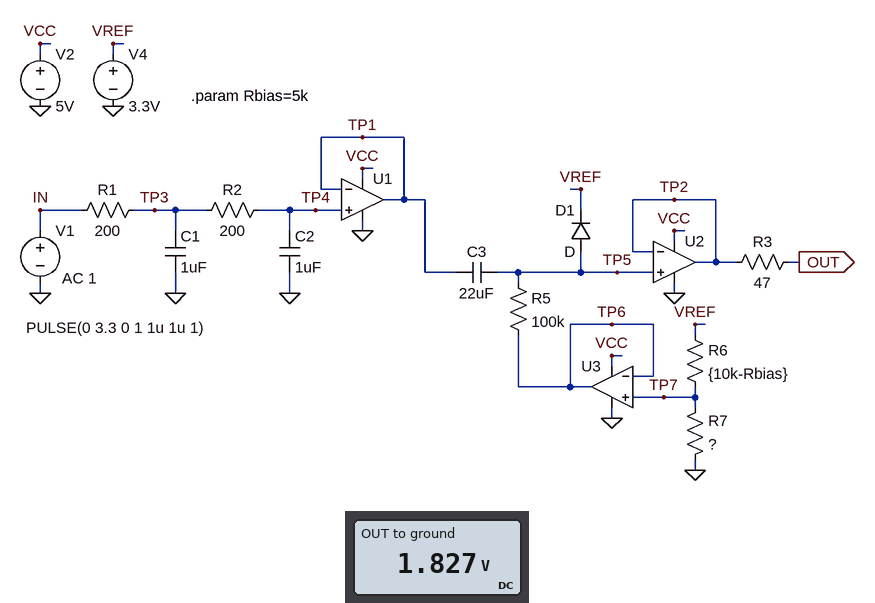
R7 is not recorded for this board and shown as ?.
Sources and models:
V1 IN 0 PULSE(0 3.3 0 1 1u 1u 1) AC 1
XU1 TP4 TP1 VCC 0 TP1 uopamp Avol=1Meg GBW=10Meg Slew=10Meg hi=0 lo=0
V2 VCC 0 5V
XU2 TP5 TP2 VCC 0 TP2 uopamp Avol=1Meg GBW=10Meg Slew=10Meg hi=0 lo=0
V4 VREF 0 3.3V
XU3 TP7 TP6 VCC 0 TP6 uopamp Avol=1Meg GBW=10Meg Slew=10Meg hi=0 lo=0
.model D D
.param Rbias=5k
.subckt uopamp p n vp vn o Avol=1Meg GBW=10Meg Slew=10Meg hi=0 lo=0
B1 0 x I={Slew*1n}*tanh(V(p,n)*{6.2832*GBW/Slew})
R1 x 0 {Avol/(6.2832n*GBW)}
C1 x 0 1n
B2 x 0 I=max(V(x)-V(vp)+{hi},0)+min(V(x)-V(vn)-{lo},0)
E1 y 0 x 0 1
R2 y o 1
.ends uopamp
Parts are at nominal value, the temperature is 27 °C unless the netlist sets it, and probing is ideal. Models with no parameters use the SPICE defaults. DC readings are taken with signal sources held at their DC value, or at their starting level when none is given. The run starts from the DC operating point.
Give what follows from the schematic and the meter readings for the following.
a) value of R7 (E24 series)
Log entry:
6.2 kΩ
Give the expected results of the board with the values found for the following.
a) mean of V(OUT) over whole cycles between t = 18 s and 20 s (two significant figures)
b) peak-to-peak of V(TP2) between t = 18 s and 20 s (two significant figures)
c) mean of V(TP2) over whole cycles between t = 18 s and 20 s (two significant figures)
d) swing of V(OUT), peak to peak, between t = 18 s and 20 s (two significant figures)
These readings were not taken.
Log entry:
1.8 V
3.3 V
1.8 V
3.3 V
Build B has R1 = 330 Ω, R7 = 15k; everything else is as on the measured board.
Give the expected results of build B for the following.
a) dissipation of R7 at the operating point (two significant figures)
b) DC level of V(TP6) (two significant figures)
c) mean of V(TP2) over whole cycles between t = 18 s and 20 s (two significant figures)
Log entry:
410 µW
2.5 V
2.4 V
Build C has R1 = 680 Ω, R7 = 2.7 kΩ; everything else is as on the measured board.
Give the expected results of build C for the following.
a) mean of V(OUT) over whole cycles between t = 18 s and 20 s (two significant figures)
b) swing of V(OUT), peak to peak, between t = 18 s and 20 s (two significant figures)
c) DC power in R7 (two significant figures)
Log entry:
1.2 V
2.7 V
500 µW
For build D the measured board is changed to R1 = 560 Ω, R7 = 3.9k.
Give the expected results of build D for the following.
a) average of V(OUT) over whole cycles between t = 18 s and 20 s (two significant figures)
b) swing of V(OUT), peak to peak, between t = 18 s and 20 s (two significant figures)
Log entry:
1.5 V
3.0 V
